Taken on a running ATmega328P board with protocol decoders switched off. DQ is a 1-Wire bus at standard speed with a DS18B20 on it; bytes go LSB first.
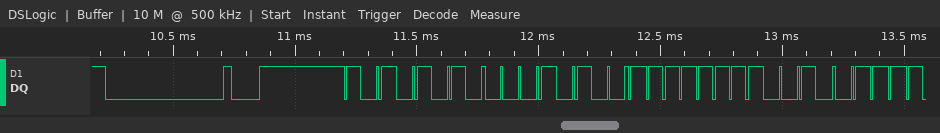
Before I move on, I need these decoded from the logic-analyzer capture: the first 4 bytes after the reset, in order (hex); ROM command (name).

55 28 FF E4
Match ROM
